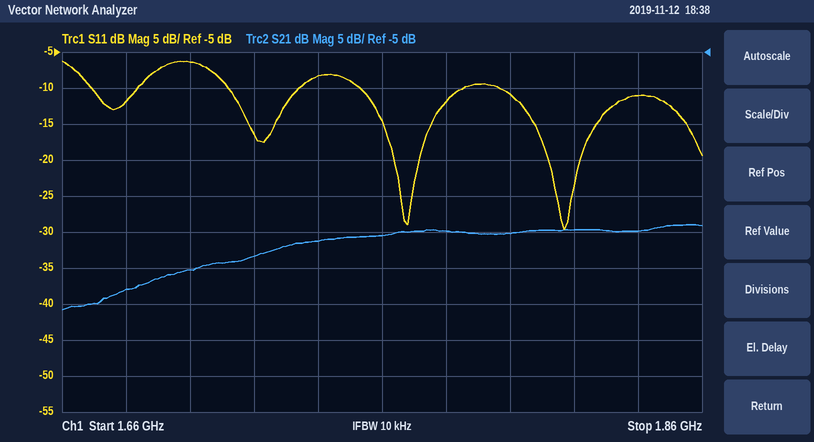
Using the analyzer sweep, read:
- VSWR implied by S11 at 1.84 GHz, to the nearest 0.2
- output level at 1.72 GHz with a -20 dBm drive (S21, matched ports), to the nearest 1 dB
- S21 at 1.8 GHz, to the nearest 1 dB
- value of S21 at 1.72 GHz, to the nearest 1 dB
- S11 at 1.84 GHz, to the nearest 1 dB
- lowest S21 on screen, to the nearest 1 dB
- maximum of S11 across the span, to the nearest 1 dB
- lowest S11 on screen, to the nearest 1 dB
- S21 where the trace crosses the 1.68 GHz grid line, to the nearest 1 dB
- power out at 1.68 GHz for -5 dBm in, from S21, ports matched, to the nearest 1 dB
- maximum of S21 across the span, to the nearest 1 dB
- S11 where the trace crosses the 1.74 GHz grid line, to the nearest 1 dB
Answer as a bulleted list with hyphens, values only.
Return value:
- 1.8
- -53 dBm
- -30 dB
- -33 dB
- -11 dB
- -41 dB
- -6 dB
- -30 dB
- -38 dB
- -43 dBm
- -29 dB
- -8 dB
